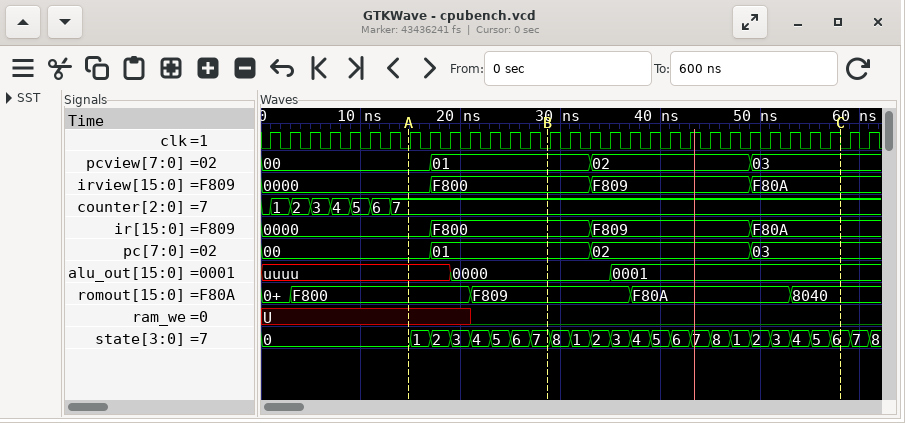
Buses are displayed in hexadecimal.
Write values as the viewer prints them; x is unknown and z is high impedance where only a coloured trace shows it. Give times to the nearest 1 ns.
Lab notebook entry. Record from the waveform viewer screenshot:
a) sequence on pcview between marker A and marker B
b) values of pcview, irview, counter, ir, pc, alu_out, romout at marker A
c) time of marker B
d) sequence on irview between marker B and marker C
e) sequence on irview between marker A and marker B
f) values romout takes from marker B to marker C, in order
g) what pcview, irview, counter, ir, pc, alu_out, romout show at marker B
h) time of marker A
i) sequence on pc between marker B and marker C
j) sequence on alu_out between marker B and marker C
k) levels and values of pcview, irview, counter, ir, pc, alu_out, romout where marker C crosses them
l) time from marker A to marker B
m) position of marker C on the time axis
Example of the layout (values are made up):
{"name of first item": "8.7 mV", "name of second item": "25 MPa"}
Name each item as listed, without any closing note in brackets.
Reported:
{"sequence on pcview between marker A and marker B": "00, 01", "values of pcview, irview, counter, ir, pc, alu_out, romout at marker A": "pcview=00, irview=0000, counter=7, ir=0000, pc=00, alu_out=uuuu, romout=F800", "time of marker B": "29 ns", "sequence on irview between marker B and marker C": "F800, F809, F80A", "sequence on irview between marker A and marker B": "0000, F800", "values romout takes from marker B to marker C, in order": "F809, F80A, 8040", "what pcview, irview, counter, ir, pc, alu_out, romout show at marker B": "pcview=01, irview=F800, counter=7, ir=F800, pc=01, alu_out=0000, romout=F809", "time of marker A": "15 ns", "sequence on pc between marker B and marker C": "01, 02, 03", "sequence on alu_out between marker B and marker C": "0000, 0001", "levels and values of pcview, irview, counter, ir, pc, alu_out, romout where marker C crosses them": "pcview=03, irview=F80A, counter=7, ir=F80A, pc=03, alu_out=0001, romout=8040", "time from marker A to marker B": "14 ns", "position of marker C on the time axis": "58 ns"}
